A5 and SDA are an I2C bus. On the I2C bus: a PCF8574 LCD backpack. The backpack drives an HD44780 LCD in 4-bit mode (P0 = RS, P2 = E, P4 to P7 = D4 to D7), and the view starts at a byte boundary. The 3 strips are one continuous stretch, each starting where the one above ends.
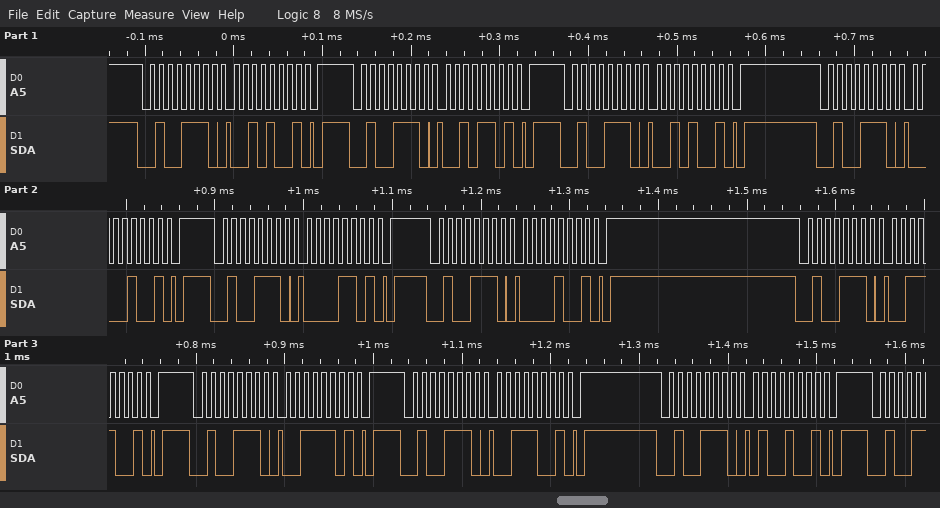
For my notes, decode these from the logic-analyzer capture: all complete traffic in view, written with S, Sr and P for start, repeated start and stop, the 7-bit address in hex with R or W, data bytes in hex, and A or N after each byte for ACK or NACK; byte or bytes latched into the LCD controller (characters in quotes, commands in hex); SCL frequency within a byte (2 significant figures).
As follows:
S 27W A 29 A P S 27W A 2D A P S 27W A 29 A P S 27W A 09 A P S 27W A 0D A P S 27W A 09 A P S 27W A 39 A P S 27W A 3D A P S 27W A 39 A P S 27W A 49 A P
' '
100 kHz
